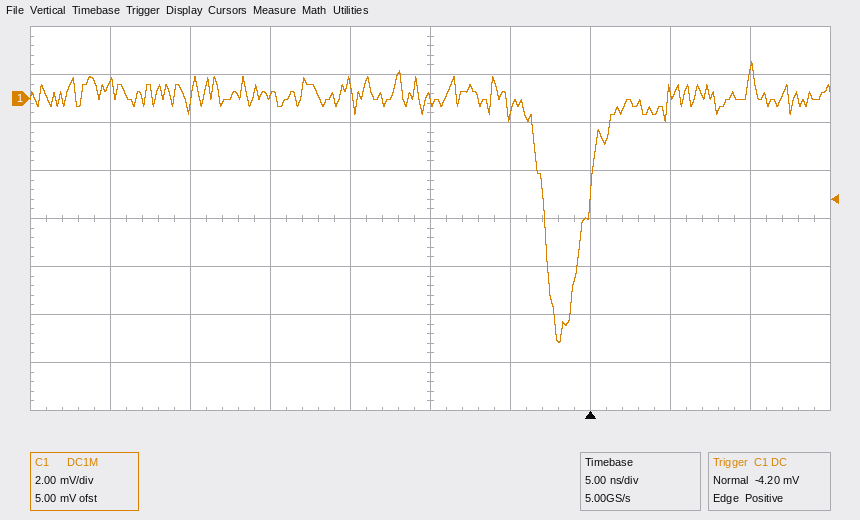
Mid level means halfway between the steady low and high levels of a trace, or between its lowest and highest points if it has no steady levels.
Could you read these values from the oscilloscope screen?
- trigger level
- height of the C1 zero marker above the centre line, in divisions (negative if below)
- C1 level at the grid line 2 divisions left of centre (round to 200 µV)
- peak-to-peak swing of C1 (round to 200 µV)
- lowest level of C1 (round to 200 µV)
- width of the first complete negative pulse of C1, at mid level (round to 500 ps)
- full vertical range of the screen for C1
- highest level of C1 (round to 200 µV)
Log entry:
-4.20 mV
+2.5 div
200 µV
11.8 mV
-10.2 mV
3.0 ns
16 mV
1.6 mV
